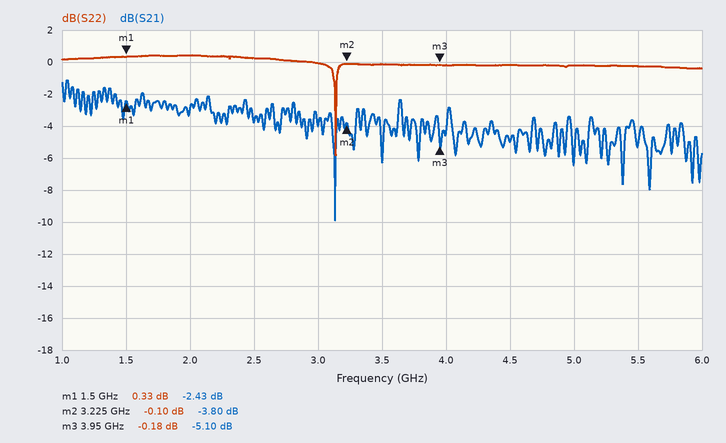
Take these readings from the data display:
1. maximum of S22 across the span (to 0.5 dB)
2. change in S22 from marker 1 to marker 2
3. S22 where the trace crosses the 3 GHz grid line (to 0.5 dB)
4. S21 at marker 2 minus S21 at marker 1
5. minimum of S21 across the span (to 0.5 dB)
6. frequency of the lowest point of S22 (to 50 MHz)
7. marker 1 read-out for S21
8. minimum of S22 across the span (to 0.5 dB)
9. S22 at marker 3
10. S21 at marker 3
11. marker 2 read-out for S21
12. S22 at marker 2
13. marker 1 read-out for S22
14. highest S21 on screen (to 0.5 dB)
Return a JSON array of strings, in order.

["0.5 dB", "-0.43 dB", "0.0 dB", "-1.37 dB", "-10.0 dB", "3.15 GHz", "-2.43 dB", "-6.0 dB", "-0.18 dB", "-5.10 dB", "-3.80 dB", "-0.10 dB", "0.33 dB", "-1.0 dB"]
